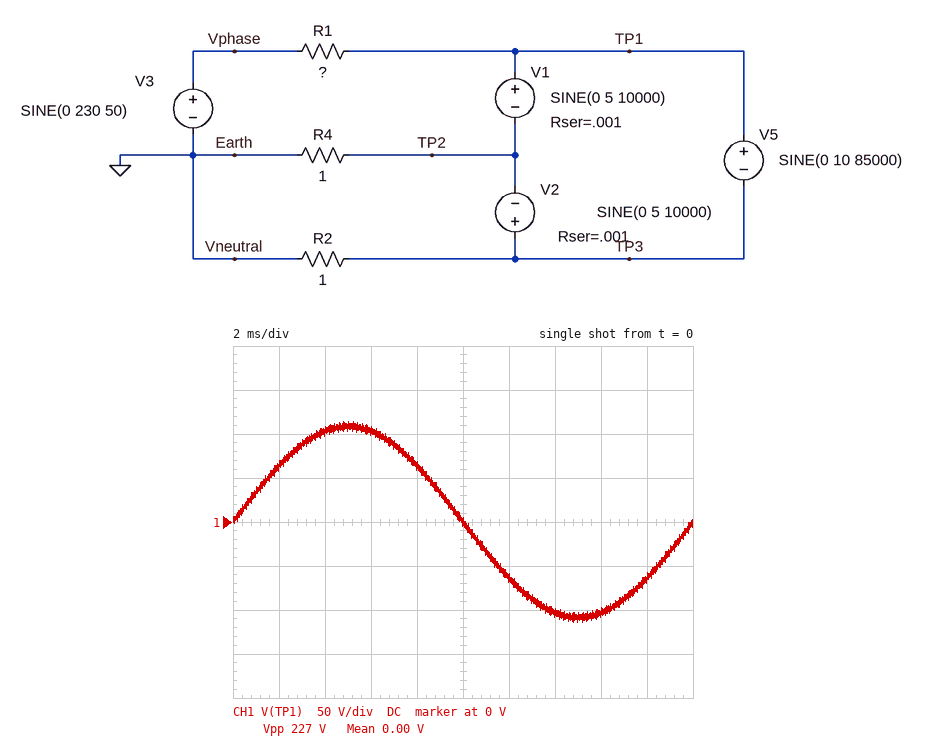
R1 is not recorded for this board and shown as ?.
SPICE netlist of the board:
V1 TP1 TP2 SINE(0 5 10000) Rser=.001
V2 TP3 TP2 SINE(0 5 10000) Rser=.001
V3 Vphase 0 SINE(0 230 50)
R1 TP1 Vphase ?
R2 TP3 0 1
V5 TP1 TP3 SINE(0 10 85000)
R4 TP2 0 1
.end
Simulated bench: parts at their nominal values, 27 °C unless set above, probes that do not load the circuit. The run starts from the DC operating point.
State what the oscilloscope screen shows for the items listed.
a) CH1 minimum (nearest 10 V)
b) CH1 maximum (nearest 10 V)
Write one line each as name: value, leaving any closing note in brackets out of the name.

CH1 minimum: -110 V
CH1 maximum: 110 V
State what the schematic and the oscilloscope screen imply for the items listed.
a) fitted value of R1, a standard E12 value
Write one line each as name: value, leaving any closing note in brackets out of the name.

fitted value of R1, a standard E12 value: 0.56 Ω
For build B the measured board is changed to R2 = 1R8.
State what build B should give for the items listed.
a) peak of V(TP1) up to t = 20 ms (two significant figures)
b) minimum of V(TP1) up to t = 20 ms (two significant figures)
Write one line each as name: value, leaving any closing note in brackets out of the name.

peak of V(TP1) up to t = 20 ms: 130 V
minimum of V(TP1) up to t = 20 ms: -130 V
